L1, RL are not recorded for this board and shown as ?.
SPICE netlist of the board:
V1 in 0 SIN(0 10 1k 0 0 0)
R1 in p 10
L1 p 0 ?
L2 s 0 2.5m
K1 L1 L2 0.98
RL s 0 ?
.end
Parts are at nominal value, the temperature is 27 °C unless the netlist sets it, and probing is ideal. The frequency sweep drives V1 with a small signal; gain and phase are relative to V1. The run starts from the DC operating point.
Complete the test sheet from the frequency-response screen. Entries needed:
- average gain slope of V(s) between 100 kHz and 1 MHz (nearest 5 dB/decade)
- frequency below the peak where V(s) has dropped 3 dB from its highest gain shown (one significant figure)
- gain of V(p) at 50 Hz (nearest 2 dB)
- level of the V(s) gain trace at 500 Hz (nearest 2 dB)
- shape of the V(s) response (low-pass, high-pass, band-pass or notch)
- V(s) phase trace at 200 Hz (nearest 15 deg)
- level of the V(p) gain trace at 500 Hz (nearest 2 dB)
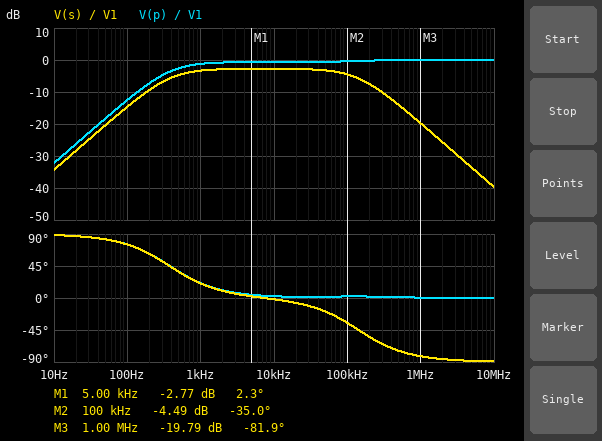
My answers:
-15 dB/decade
400 Hz
-18 dB
-4 dB
band-pass
60 deg
-2 dB
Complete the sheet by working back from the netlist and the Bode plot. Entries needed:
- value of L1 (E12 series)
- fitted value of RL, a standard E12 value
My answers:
3.9 mH
82 Ω
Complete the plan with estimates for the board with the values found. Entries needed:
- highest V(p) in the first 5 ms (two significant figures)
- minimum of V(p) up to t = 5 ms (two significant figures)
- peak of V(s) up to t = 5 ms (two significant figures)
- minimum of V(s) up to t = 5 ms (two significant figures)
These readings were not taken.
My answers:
8.7 V
-9.3 V
6.8 V
-7.3 V
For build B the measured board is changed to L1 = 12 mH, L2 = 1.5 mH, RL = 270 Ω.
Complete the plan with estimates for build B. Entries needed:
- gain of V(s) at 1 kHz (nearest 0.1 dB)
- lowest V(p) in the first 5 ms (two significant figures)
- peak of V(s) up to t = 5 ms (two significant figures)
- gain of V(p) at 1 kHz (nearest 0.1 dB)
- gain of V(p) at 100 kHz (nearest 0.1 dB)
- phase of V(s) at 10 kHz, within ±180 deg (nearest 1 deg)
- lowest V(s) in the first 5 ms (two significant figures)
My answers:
-9.3 dB
-11 V
3.4 V
-0.1 dB
0 dB
0 deg
-3.7 V
